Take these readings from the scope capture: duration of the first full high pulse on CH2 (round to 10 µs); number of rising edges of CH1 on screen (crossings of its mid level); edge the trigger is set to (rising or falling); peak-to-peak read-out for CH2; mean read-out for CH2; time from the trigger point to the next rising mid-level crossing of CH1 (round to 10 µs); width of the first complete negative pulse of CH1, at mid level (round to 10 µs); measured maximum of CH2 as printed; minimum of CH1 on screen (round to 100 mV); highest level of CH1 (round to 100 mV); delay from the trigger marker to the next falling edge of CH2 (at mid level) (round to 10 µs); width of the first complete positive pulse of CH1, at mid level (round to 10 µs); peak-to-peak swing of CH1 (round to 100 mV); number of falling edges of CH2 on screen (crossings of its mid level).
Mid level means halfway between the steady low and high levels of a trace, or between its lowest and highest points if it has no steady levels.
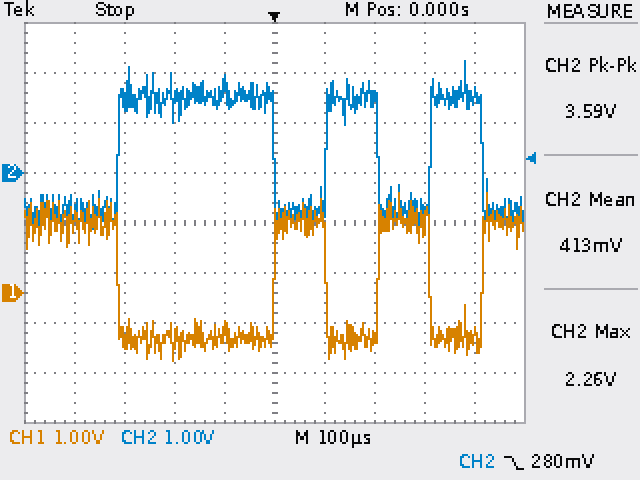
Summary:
310 µs
3
falling
3.59 V
413 mV
210 µs
310 µs
2.26 V
-1.4 V
2.0 V
210 µs
100 µs
3.4 V
3
